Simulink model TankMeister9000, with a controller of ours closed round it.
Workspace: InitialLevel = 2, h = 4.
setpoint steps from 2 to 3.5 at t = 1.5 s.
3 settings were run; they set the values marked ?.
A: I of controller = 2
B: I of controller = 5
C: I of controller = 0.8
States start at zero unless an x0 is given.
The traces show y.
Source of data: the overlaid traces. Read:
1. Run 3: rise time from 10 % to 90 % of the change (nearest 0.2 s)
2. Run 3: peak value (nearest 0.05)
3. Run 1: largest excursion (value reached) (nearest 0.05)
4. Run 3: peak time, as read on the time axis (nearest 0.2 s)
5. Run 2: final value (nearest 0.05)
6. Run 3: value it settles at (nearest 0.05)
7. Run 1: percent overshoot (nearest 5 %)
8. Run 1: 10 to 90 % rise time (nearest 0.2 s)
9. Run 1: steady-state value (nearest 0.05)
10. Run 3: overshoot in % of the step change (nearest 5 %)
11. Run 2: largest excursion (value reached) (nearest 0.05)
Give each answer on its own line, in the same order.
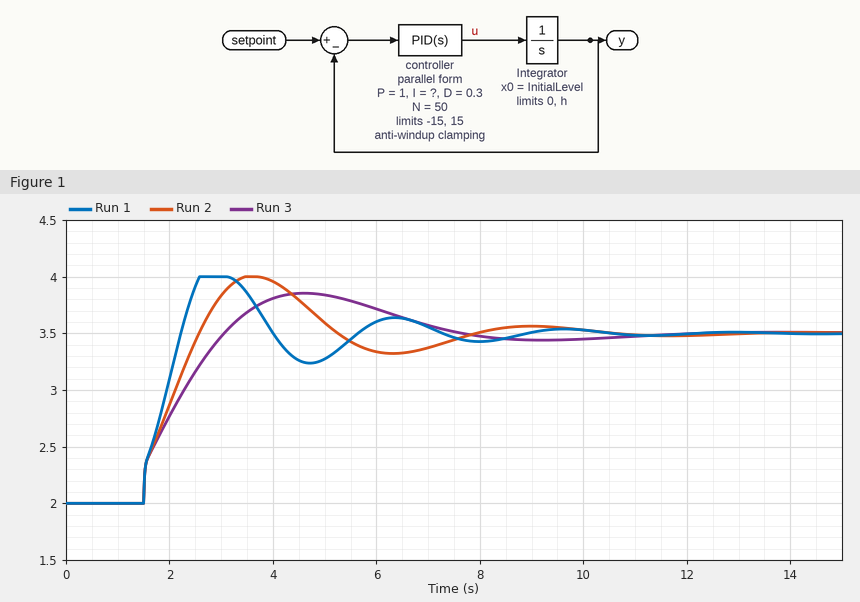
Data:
1.2 s
3.85
4.00
4.6 s
3.50
3.50
35 %
0.6 s
3.50
25 %
4.00
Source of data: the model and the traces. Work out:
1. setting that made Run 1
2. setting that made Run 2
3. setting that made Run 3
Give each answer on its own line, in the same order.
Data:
B
A
C
